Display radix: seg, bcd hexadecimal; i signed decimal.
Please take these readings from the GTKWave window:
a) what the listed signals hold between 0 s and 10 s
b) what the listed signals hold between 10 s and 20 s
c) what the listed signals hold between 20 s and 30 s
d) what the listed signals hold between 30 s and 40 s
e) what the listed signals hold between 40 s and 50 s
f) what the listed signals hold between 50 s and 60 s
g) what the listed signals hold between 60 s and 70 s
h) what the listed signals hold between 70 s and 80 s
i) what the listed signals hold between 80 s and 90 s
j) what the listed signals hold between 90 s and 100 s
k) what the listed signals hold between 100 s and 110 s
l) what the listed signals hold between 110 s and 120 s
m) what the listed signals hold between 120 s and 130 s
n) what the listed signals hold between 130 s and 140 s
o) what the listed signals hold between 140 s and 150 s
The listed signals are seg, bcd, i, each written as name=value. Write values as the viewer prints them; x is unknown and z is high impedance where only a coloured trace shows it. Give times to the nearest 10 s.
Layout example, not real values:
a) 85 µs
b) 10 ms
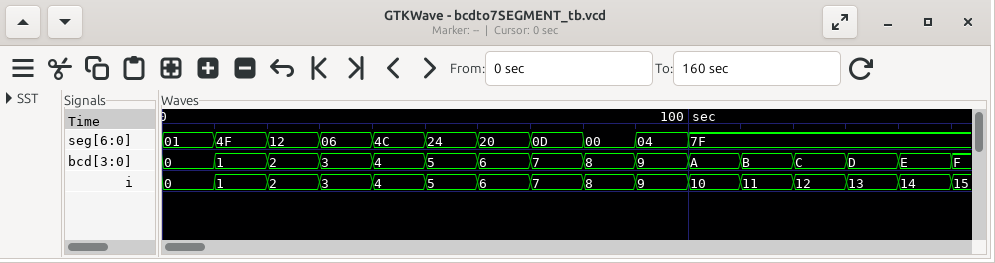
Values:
a) seg=01, bcd=0, i=0
b) seg=4F, bcd=1, i=1
c) seg=12, bcd=2, i=2
d) seg=06, bcd=3, i=3
e) seg=4C, bcd=4, i=4
f) seg=24, bcd=5, i=5
g) seg=20, bcd=6, i=6
h) seg=0D, bcd=7, i=7
i) seg=00, bcd=8, i=8
j) seg=04, bcd=9, i=9
k) seg=7F, bcd=A, i=10
l) seg=7F, bcd=B, i=11
m) seg=7F, bcd=C, i=12
n) seg=7F, bcd=D, i=13
o) seg=7F, bcd=E, i=14
